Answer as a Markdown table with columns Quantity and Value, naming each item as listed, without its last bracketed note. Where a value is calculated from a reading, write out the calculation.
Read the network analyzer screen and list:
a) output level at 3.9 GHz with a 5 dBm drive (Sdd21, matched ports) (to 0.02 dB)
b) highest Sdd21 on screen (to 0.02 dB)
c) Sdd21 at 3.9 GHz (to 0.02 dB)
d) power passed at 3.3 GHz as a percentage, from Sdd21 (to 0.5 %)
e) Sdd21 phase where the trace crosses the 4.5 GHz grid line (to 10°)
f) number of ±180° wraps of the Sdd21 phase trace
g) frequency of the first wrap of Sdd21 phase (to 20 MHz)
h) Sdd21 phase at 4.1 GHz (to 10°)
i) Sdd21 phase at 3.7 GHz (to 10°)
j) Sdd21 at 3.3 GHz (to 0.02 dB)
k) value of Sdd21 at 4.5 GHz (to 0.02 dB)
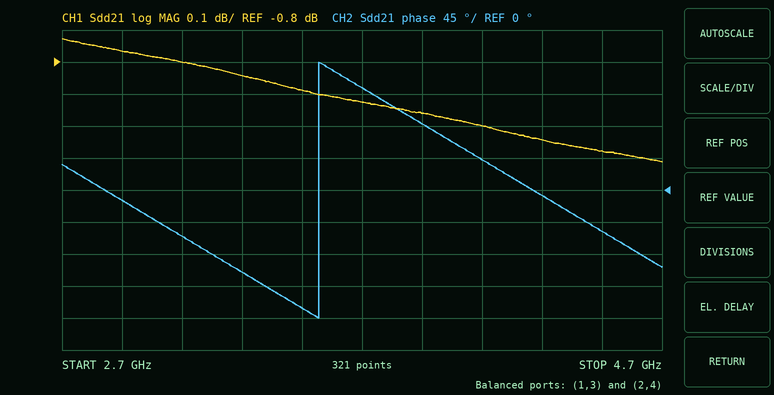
| Quantity | Value |
|---|---|
| output level at 3.9 GHz with a 5 dBm drive (Sdd21, matched ports) | 5 dBm + (-0.96 dB) = 4.04 dBm |
| highest Sdd21 on screen | -0.72 dB |
| Sdd21 at 3.9 GHz | -0.96 dB |
| power passed at 3.3 GHz as a percentage, from Sdd21 | 10^(-0.84/10) ≈ 82.4 %, so 82.5 % to the nearest 0.5 % |
| Sdd21 phase where the trace crosses the 4.5 GHz grid line | -60° |
| number of ±180° wraps of the Sdd21 phase trace | 1 |
| frequency of the first wrap of Sdd21 phase | 3.56 GHz |
| Sdd21 phase at 4.1 GHz | 40° |
| Sdd21 phase at 3.7 GHz | 140° |
| Sdd21 at 3.3 GHz | -0.84 dB |
| value of Sdd21 at 4.5 GHz | -1.08 dB |
